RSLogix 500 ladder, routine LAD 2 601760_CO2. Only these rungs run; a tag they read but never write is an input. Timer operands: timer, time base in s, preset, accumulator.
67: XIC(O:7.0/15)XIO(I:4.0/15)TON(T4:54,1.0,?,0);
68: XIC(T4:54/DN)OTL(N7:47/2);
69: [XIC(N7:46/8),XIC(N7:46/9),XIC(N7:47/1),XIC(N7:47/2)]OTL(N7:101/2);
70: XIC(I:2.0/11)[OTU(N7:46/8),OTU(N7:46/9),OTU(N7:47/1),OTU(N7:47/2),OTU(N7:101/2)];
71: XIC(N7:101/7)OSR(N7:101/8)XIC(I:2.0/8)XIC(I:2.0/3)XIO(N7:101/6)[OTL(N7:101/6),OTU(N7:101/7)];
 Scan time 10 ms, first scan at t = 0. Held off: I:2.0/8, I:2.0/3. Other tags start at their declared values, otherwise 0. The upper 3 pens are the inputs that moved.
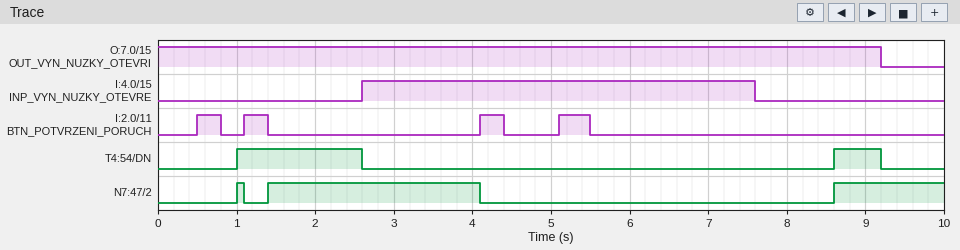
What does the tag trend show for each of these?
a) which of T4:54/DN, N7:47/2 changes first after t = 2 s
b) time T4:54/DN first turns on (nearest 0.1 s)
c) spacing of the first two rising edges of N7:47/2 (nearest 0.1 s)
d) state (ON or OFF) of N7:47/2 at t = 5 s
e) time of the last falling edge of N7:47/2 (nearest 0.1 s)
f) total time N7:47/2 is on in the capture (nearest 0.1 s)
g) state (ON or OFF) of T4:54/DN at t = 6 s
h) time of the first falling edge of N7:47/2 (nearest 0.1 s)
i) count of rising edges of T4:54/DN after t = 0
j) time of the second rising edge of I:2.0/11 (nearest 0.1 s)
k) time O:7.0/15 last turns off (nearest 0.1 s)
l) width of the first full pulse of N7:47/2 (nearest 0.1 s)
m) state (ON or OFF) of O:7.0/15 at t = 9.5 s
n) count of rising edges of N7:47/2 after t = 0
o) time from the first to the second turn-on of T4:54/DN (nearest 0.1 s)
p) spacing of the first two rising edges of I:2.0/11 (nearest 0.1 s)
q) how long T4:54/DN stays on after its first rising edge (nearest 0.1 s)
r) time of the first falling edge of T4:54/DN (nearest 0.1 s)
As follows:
T4:54/DN
1.0 s
0.4 s
OFF
4.1 s
4.2 s
OFF
1.1 s
2
1.1 s
9.2 s
0.1 s
OFF
3
7.6 s
0.6 s
1.6 s
2.6 s
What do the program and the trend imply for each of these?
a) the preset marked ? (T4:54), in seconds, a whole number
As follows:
1 s
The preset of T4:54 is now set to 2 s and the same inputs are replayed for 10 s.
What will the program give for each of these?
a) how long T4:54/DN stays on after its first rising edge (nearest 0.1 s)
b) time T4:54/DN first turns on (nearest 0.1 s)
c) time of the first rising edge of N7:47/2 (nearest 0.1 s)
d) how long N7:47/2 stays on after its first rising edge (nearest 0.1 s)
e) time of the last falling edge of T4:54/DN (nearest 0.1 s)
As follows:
0.6 s
2.0 s
2.0 s
2.1 s
2.6 s
